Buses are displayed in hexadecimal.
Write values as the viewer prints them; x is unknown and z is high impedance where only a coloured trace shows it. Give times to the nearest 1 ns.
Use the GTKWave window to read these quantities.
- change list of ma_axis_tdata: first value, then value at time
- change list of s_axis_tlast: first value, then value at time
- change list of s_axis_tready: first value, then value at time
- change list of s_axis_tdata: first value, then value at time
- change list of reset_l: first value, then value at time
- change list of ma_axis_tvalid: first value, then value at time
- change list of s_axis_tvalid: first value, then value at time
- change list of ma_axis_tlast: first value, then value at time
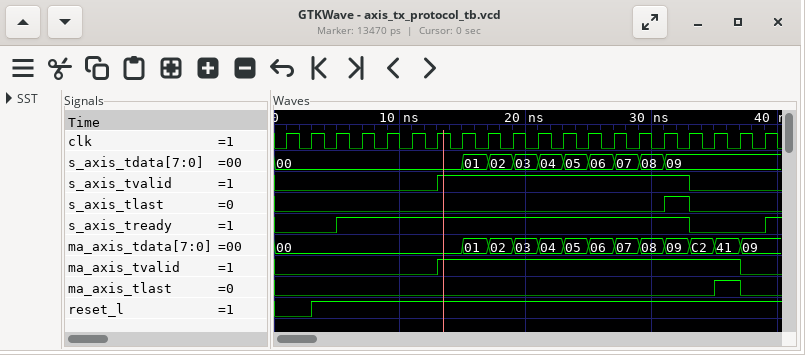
00, 01 at 15 ns, 02 at 17 ns, 03 at 19 ns, 04 at 21 ns, 05 at 23 ns, 06 at 25 ns, 07 at 27 ns, 08 at 29 ns, 09 at 31 ns, C2 at 33 ns, 41 at 35 ns, 09 at 37 ns
0, 1 at 31 ns, 0 at 33 ns
0, 1 at 5 ns, 0 at 33 ns, 1 at 39 ns
00, 01 at 15 ns, 02 at 17 ns, 03 at 19 ns, 04 at 21 ns, 05 at 23 ns, 06 at 25 ns, 07 at 27 ns, 08 at 29 ns, 09 at 31 ns
0, 1 at 3 ns
0, 1 at 13 ns, 0 at 37 ns
0, 1 at 13 ns, 0 at 33 ns
0, 1 at 35 ns, 0 at 37 ns
